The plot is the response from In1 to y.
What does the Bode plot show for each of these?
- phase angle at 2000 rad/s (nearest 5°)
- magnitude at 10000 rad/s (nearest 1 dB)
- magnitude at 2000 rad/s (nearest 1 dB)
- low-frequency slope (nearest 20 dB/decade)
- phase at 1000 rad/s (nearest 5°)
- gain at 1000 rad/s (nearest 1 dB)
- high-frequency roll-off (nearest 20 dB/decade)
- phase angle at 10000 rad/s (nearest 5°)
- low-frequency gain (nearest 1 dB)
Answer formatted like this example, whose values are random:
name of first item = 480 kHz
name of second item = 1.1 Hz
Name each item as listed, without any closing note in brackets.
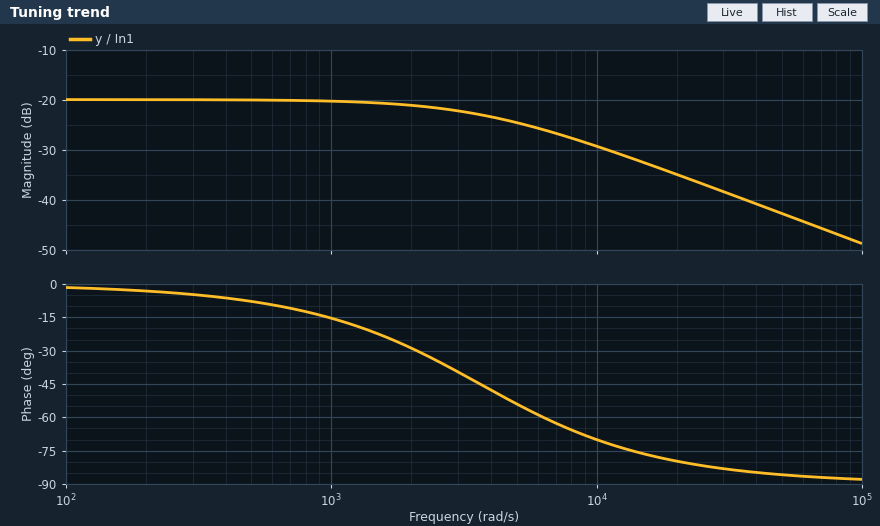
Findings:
phase angle at 2000 rad/s = -30°
magnitude at 10000 rad/s = -29 dB
magnitude at 2000 rad/s = -21 dB
low-frequency slope = 0 dB/decade
phase at 1000 rad/s = -15°
gain at 1000 rad/s = -20 dB
high-frequency roll-off = -20 dB/decade
phase angle at 10000 rad/s = -70°
low-frequency gain = -20 dB
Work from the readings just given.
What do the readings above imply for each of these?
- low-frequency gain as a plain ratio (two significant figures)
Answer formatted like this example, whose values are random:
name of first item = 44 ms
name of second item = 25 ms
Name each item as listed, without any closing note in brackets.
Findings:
low-frequency gain as a plain ratio = 0.10
